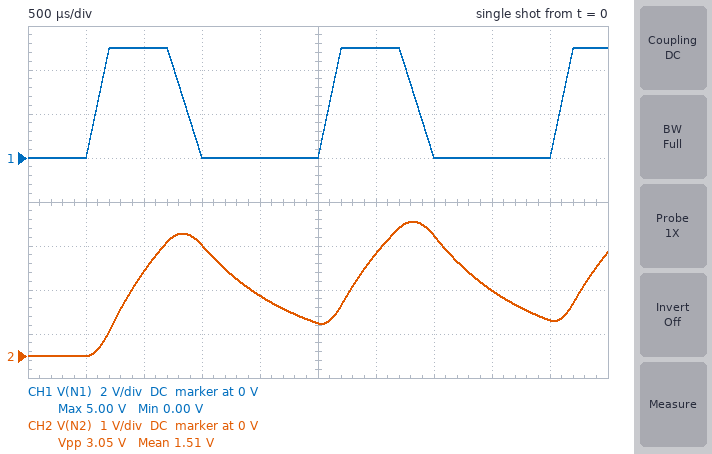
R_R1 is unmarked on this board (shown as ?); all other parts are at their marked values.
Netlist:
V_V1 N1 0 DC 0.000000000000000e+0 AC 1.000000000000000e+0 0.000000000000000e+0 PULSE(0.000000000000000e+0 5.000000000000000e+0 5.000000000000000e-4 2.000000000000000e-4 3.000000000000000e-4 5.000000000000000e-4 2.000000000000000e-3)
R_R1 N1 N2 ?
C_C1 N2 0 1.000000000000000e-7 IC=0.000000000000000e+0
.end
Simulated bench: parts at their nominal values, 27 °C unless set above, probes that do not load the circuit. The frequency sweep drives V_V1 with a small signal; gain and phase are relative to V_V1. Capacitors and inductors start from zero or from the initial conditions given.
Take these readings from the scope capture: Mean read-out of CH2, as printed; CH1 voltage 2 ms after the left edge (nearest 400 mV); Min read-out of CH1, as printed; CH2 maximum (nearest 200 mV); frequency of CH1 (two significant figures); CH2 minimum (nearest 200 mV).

1.51 V
0 V
0.00 V
3.0 V
500 Hz
0 V
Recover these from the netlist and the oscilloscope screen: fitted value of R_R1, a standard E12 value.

8.2 kΩ
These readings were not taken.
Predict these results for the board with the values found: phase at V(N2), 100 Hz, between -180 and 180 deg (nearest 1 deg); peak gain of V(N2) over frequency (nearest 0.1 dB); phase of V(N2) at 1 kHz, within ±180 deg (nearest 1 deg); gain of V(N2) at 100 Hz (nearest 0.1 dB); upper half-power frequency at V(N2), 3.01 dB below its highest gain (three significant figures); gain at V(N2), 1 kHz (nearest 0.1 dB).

-27 deg
0 dB
-79 deg
-1.0 dB
194 Hz
-14.4 dB
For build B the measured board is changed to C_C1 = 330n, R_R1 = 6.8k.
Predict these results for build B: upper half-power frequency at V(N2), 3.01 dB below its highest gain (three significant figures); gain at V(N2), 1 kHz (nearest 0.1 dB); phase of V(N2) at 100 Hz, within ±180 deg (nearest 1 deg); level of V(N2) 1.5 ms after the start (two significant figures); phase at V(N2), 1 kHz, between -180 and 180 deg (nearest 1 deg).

70.9 Hz
-23.0 dB
-55 deg
1.3 V
-86 deg
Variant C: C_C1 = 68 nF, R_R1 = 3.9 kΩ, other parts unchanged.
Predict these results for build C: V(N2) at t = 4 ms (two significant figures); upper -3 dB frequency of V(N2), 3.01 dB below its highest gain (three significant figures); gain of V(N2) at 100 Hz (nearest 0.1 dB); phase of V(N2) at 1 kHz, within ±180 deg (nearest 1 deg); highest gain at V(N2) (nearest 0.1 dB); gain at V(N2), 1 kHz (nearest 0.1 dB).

430 mV
600 Hz
-0.1 dB
-59 deg
0 dB
-5.8 dB
